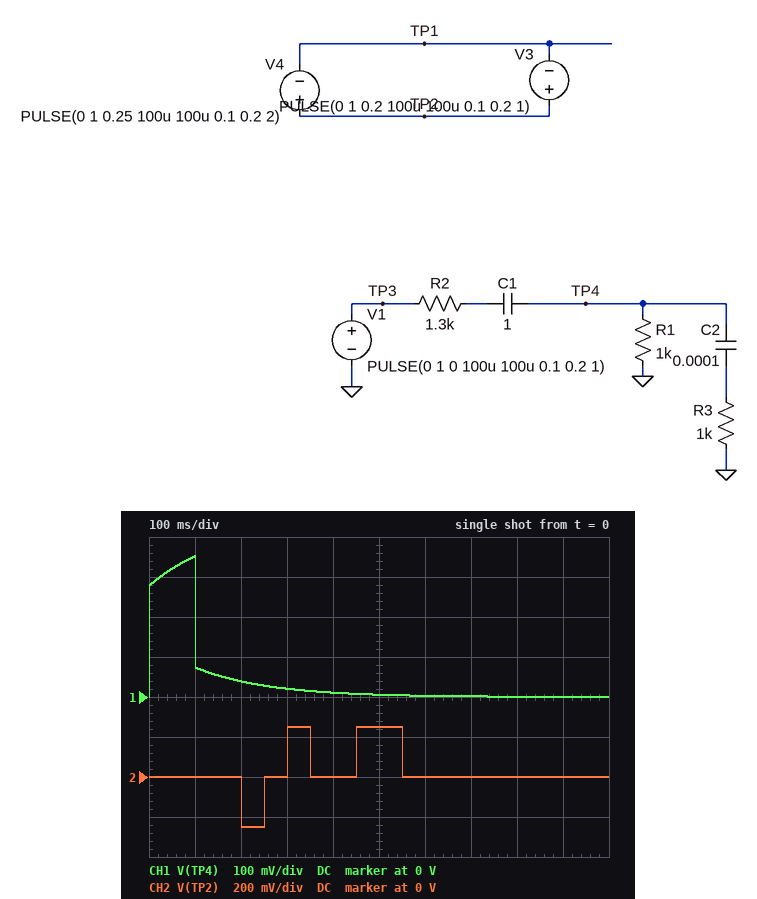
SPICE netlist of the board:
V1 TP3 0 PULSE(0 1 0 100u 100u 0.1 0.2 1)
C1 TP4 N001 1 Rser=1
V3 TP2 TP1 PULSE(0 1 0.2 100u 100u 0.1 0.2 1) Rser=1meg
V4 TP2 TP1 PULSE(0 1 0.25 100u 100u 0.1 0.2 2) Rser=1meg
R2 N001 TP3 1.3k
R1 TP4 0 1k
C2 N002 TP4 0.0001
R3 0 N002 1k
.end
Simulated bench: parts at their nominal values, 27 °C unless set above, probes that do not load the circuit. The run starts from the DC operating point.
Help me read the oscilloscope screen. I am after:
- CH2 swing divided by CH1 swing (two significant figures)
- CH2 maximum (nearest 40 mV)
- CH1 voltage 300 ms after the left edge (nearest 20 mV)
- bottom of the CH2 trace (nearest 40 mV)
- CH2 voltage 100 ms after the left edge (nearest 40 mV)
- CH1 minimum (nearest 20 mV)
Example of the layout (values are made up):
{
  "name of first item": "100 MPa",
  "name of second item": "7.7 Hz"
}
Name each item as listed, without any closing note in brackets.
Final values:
{
  "CH2 swing divided by CH1 swing": "1.4",
  "CH2 maximum": "240 mV",
  "CH1 voltage 300 ms after the left edge": "20 mV",
  "bottom of the CH2 trace": "-240 mV",
  "CH2 voltage 100 ms after the left edge": "0 V",
  "CH1 minimum": "0 V"
}
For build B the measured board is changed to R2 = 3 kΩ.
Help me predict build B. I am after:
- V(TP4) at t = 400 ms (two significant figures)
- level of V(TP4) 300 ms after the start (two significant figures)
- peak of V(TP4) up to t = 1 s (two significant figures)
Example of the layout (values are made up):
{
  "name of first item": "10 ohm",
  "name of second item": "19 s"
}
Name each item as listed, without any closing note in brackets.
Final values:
{
  "V(TP4) at t = 400 ms": "8.4 mV",
  "level of V(TP4) 300 ms after the start": "15 mV",
  "peak of V(TP4) up to t = 1 s": "190 mV"
}
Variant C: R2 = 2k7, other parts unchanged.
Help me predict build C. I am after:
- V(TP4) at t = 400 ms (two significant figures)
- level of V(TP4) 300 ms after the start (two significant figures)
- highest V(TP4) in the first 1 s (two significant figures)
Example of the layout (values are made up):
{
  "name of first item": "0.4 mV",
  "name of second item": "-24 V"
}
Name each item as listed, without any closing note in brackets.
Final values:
{
  "V(TP4) at t = 400 ms": "8.8 mV",
  "level of V(TP4) 300 ms after the start": "16 mV",
  "highest V(TP4) in the first 1 s": "210 mV"
}
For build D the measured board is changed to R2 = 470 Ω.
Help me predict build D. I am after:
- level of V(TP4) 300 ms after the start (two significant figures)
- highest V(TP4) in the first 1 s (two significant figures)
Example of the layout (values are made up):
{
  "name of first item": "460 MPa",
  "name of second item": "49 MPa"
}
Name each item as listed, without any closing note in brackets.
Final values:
{
  "level of V(TP4) 300 ms after the start": "19 mV",
  "highest V(TP4) in the first 1 s": "600 mV"
}
